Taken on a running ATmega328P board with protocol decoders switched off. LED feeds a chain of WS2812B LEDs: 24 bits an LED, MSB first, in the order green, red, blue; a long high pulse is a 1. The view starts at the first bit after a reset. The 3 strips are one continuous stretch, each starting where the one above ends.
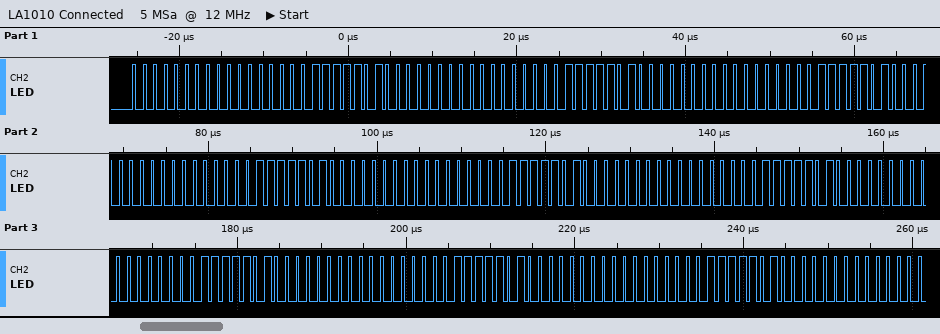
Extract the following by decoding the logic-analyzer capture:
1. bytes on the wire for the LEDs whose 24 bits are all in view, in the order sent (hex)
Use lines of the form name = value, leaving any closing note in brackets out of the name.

bytes on the wire for the LEDs whose 24 bits are all in view, in the order sent = 00 00 7D 00 00 7D 00 00 7D 00 00 7D 00 00 7D 00 00 7D 00 00 7D 00 00 7D 00 00 7D
